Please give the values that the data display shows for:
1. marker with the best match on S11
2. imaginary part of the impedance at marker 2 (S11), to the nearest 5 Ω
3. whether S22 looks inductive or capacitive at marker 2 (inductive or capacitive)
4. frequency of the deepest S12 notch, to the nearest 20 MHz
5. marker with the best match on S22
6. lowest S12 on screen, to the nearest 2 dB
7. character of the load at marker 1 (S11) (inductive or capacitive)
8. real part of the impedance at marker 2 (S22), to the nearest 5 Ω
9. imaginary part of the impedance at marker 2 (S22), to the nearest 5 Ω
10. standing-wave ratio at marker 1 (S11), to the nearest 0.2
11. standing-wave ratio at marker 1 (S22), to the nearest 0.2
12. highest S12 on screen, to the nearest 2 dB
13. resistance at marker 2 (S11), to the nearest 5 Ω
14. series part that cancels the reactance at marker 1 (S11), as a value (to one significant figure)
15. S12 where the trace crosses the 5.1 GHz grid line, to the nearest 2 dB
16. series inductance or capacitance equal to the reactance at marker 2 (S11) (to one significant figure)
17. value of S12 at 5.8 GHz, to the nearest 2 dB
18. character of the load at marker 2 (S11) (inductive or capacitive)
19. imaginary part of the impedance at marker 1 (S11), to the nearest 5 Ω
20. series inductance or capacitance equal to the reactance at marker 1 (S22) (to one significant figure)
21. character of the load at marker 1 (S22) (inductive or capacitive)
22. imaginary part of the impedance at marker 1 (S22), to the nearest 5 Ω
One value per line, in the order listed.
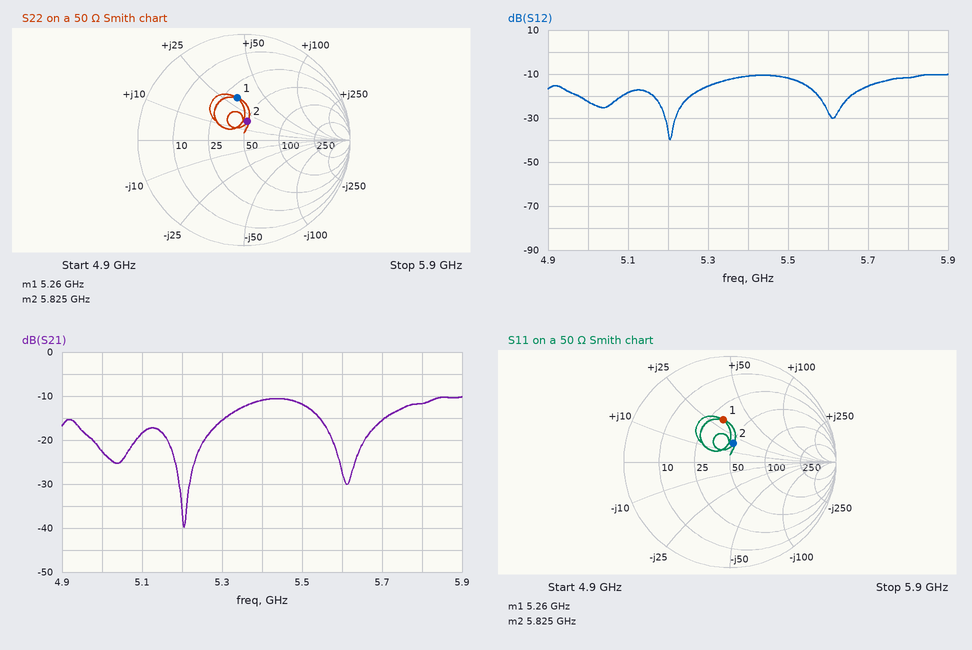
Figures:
marker 2
+20 Ω
inductive
5.20 GHz
marker 2
-40 dB
inductive
50 Ω
+20 Ω
2.4
2.4
-10 dB
50 Ω
1.0 pF
-18 dB
500 pH
-12 dB
inductive
+30 Ω
900 pH
inductive
+30 Ω
